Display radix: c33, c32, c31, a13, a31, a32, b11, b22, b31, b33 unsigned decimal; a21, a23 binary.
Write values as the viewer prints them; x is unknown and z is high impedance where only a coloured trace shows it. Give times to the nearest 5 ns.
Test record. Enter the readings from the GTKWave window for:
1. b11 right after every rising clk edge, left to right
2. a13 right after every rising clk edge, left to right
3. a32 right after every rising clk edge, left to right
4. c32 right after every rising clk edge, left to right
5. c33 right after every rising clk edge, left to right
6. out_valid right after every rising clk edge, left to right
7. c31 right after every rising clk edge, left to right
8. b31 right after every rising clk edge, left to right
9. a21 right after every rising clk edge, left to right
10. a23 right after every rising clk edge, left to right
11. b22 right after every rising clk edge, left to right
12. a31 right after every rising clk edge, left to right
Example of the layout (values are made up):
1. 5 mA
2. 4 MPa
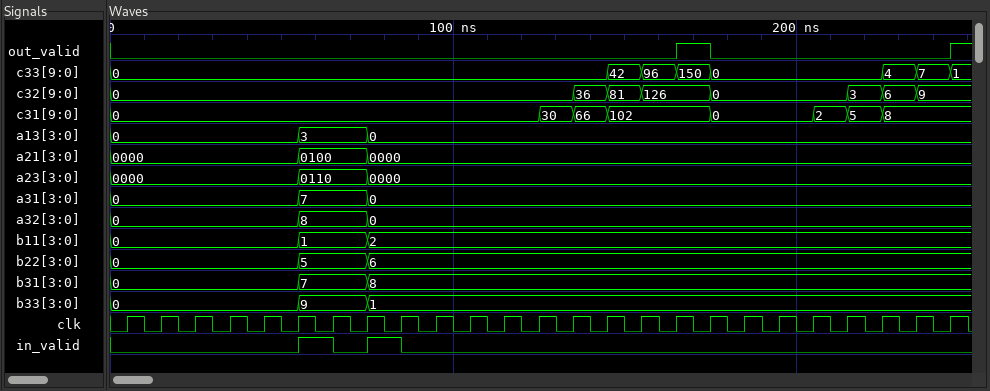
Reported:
1. 0, 0, 0, 0, 0, 1, 1, 2, 2, 2, 2, 2, 2, 2, 2, 2, 2, 2, 2, 2, 2, 2, 2, 2, 2
2. 0, 0, 0, 0, 0, 3, 3, 0, 0, 0, 0, 0, 0, 0, 0, 0, 0, 0, 0, 0, 0, 0, 0, 0, 0
3. 0, 0, 0, 0, 0, 8, 8, 0, 0, 0, 0, 0, 0, 0, 0, 0, 0, 0, 0, 0, 0, 0, 0, 0, 0
4. 0, 0, 0, 0, 0, 0, 0, 0, 0, 0, 0, 0, 0, 36, 81, 126, 126, 0, 0, 0, 0, 3, 6, 9, 9
5. 0, 0, 0, 0, 0, 0, 0, 0, 0, 0, 0, 0, 0, 0, 42, 96, 150, 0, 0, 0, 0, 0, 4, 7, 1
6. 0 0 0 0 0 0 0 0 0 0 0 0 0 0 0 0 1 0 0 0 0 0 0 0 1
7. 0, 0, 0, 0, 0, 0, 0, 0, 0, 0, 0, 0, 30, 66, 102, 102, 102, 0, 0, 0, 2, 5, 8, 8, 8
8. 0, 0, 0, 0, 0, 7, 7, 8, 8, 8, 8, 8, 8, 8, 8, 8, 8, 8, 8, 8, 8, 8, 8, 8, 8
9. 0000, 0000, 0000, 0000, 0000, 0100, 0100, 0000, 0000, 0000, 0000, 0000, 0000, 0000, 0000, 0000, 0000, 0000, 0000, 0000, 0000, 0000, 0000, 0000, 0000
10. 0000, 0000, 0000, 0000, 0000, 0110, 0110, 0000, 0000, 0000, 0000, 0000, 0000, 0000, 0000, 0000, 0000, 0000, 0000, 0000, 0000, 0000, 0000, 0000, 0000
11. 0, 0, 0, 0, 0, 5, 5, 6, 6, 6, 6, 6, 6, 6, 6, 6, 6, 6, 6, 6, 6, 6, 6, 6, 6
12. 0, 0, 0, 0, 0, 7, 7, 0, 0, 0, 0, 0, 0, 0, 0, 0, 0, 0, 0, 0, 0, 0, 0, 0, 0
